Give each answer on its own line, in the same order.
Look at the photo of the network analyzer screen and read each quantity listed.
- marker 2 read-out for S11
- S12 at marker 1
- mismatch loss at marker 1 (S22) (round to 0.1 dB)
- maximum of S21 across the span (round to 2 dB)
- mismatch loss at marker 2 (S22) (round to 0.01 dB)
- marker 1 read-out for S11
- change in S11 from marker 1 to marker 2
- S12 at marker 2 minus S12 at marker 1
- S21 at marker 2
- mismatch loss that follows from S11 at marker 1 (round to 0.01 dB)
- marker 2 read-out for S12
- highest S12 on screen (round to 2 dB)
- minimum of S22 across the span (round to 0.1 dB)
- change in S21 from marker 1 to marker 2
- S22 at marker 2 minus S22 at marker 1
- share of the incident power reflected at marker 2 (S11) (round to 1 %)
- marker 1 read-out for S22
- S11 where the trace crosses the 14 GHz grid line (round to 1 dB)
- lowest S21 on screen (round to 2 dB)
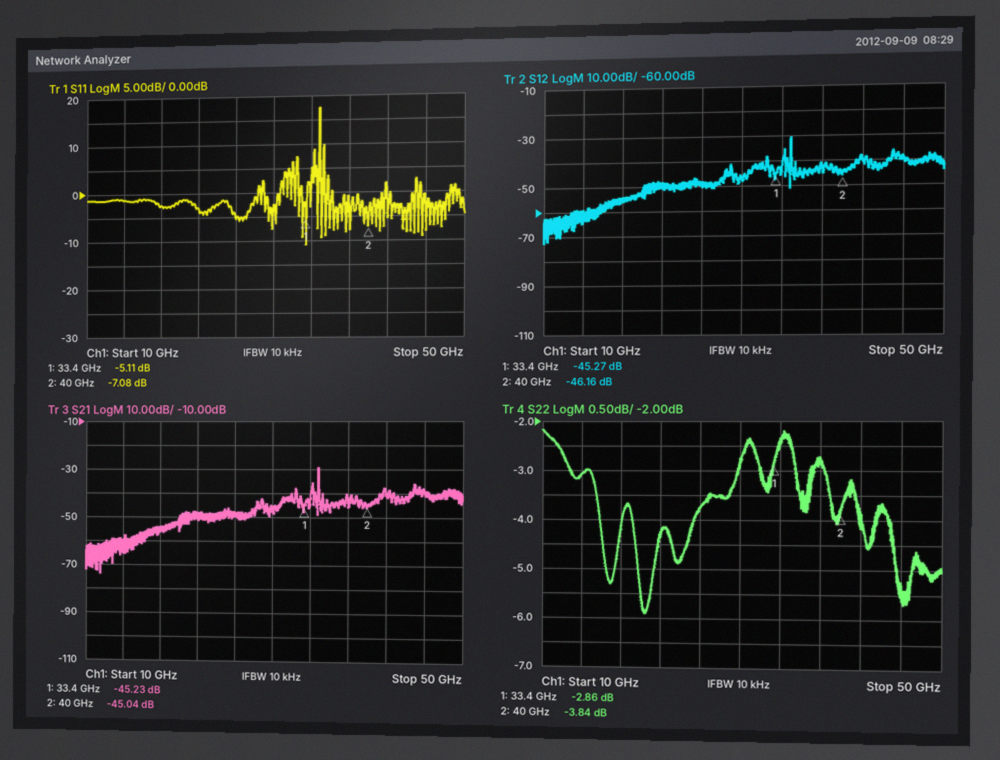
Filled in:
-7.08 dB
-45.27 dB
3.2 dB
-30 dB
2.31 dB
-5.11 dB
-1.97 dB
-0.89 dB
-45.04 dB
1.60 dB
-46.16 dB
-30 dB
-5.9 dB
0.19 dB
-0.98 dB
20 %
-2.86 dB
-1 dB
-74 dB
